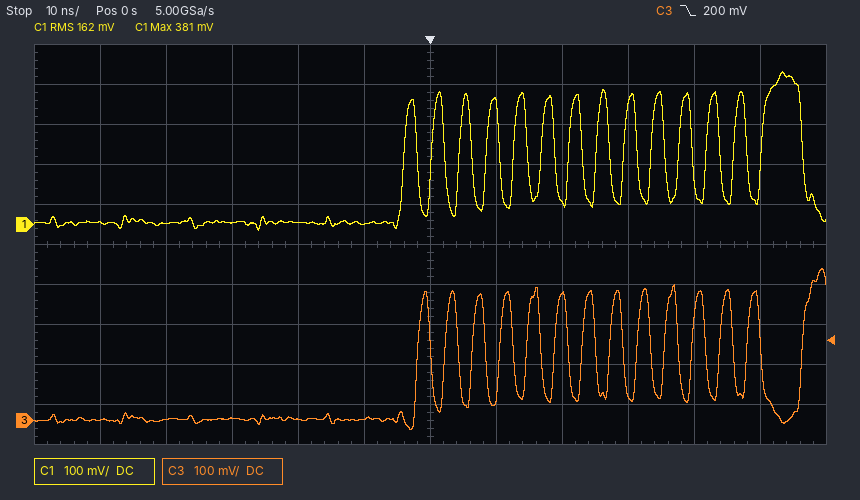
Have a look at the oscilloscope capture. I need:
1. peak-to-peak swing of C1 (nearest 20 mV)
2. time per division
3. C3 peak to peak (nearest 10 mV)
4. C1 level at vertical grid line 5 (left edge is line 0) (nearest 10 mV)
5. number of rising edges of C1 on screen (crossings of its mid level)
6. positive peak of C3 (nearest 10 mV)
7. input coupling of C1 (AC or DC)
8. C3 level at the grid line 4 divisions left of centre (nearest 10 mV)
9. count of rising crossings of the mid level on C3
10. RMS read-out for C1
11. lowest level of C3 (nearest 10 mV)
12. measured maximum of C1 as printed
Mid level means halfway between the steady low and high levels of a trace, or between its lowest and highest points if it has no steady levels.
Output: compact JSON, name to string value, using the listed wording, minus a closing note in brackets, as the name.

{"peak-to-peak swing of C1": "400 mV", "time per division": "10 ns", "C3 peak to peak": "400 mV", "C1 level at vertical grid line 5 (left edge is line 0)": "0 mV", "number of rising edges of C1 on screen": "14", "positive peak of C3": "380 mV", "input coupling of C1": "DC", "C3 level at the grid line 4 divisions left of centre": "0 mV", "count of rising crossings of the mid level on C3": "14", "RMS read-out for C1": "162 mV", "lowest level of C3": "-20 mV", "measured maximum of C1 as printed": "381 mV"}
